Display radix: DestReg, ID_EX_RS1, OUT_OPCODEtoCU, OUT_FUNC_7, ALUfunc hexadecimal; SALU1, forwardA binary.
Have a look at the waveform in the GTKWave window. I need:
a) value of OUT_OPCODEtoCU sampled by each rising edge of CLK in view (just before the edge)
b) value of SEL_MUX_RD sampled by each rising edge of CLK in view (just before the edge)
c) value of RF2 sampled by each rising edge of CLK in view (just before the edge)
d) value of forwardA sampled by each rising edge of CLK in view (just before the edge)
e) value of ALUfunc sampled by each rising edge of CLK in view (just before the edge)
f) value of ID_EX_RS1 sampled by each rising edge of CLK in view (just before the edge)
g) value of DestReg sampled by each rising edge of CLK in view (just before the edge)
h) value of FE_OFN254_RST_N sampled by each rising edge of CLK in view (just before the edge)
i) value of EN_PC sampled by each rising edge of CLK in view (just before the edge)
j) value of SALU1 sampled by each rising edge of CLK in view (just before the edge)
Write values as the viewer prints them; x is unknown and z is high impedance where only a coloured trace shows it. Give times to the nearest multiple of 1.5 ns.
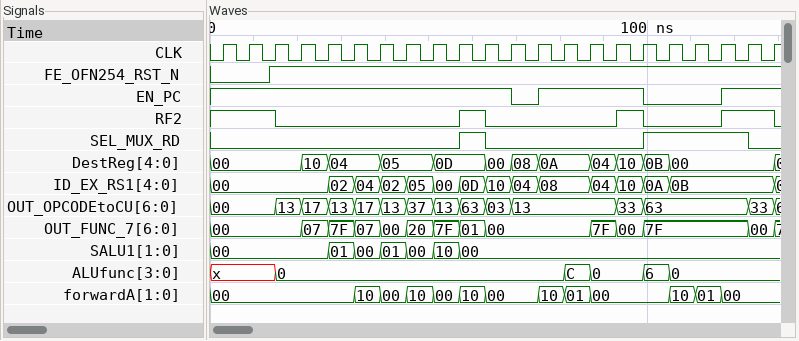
00, 00, 00, 13, 17, 13, 17, 13, 37, 13, 63, 03, 13, 13, 13, 13, 33, 63, 63, 63, 63, 33
0 0 0 0 0 0 0 0 0 0 1 0 0 0 0 0 0 1 1 1 1 0
1 1 1 0 0 0 0 0 0 0 1 0 0 0 0 0 1 0 0 0 1 1
00, 00, 00, 00, 00, 00, 10, 00, 10, 00, 10, 00, 00, 10, 01, 00, 00, 00, 10, 01, 00, 00
x, x, x, 0, 0, 0, 0, 0, 0, 0, 0, 0, 0, 0, C, 0, 0, 6, 0, 0, 0, 0
00, 00, 00, 00, 00, 02, 04, 02, 05, 00, 0D, 10, 04, 08, 08, 04, 10, 0A, 0B, 0B, 0B, 0B
00, 00, 00, 00, 10, 04, 04, 05, 05, 0D, 0D, 00, 08, 0A, 0A, 04, 10, 0B, 00, 00, 00, 00
0 0 1 1 1 1 1 1 1 1 1 1 1 1 1 1 1 1 1 1 1 1
1 1 1 1 1 1 1 1 1 1 1 1 0 1 1 1 1 0 0 0 1 1
00, 00, 00, 00, 00, 01, 00, 01, 00, 10, 00, 00, 00, 00, 00, 00, 00, 00, 00, 00, 00, 00
